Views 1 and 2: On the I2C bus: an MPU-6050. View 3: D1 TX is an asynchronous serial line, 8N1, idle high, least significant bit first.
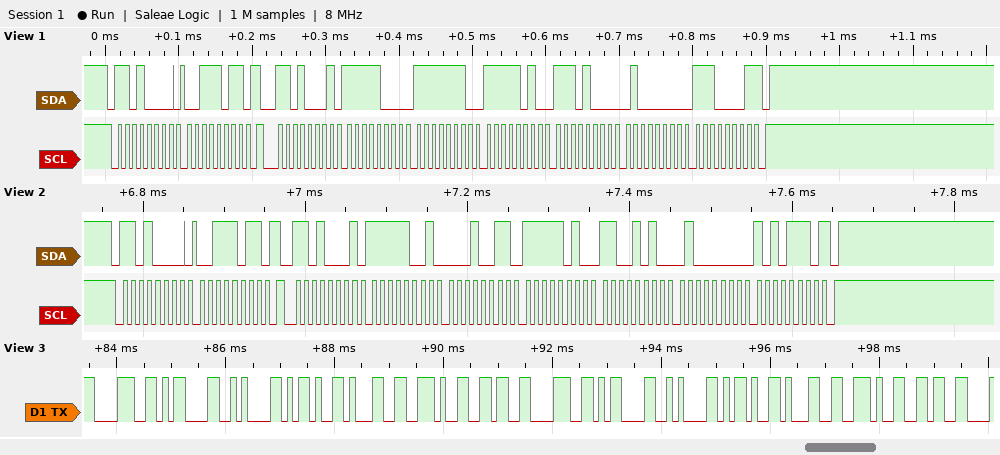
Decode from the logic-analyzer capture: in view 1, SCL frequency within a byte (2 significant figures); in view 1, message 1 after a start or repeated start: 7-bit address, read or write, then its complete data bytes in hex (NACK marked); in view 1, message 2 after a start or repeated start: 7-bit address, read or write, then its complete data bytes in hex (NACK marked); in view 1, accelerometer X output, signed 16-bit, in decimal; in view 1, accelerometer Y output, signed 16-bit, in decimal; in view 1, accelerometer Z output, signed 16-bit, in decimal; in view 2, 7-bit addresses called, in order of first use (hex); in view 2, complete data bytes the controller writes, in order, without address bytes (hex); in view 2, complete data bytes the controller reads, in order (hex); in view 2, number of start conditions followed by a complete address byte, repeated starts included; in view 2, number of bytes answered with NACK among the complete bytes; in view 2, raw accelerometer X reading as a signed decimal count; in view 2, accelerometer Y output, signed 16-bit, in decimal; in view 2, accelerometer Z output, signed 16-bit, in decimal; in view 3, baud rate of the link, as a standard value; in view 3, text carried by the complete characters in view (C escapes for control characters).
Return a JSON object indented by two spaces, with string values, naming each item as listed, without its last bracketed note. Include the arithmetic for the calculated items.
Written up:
{
  "in view 1, SCL frequency within a byte": "100 kHz",
  "in view 1, message 1 after a start or repeated start: 7-bit address, read or write, then its complete data bytes in hex": "0x68 write: 3B",
  "in view 1, message 2 after a start or repeated start: 7-bit address, read or write, then its complete data bytes in hex": "0x68 read: F8 FE FA E8 40 E1 NACK",
  "in view 1, accelerometer X output, signed 16-bit, in decimal": "0xF8FE = -1794",
  "in view 1, accelerometer Y output, signed 16-bit, in decimal": "0xFAE8 = -1304",
  "in view 1, accelerometer Z output, signed 16-bit, in decimal": "0x40E1 = 16609",
  "in view 2, 7-bit addresses called, in order of first use": "0x68",
  "in view 2, complete data bytes the controller writes, in order, without address bytes": "3B",
  "in view 2, complete data bytes the controller reads, in order": "F9 13 FA CA 40 AE",
  "in view 2, number of start conditions followed by a complete address byte, repeated starts included": "2",
  "in view 2, number of bytes answered with NACK among the complete bytes": "1",
  "in view 2, raw accelerometer X reading as a signed decimal count": "0xF913 = -1773",
  "in view 2, accelerometer Y output, signed 16-bit, in decimal": "0xFACA = -1334",
  "in view 2, accelerometer Z output, signed 16-bit, in decimal": "0x40AE = 16558",
  "in view 3, baud rate of the link, as a standard value": "9600 baud",
  "in view 3, text carried by the complete characters in view": "\"8\\r\\n-1.68\\r\\n-1.6\""
}
